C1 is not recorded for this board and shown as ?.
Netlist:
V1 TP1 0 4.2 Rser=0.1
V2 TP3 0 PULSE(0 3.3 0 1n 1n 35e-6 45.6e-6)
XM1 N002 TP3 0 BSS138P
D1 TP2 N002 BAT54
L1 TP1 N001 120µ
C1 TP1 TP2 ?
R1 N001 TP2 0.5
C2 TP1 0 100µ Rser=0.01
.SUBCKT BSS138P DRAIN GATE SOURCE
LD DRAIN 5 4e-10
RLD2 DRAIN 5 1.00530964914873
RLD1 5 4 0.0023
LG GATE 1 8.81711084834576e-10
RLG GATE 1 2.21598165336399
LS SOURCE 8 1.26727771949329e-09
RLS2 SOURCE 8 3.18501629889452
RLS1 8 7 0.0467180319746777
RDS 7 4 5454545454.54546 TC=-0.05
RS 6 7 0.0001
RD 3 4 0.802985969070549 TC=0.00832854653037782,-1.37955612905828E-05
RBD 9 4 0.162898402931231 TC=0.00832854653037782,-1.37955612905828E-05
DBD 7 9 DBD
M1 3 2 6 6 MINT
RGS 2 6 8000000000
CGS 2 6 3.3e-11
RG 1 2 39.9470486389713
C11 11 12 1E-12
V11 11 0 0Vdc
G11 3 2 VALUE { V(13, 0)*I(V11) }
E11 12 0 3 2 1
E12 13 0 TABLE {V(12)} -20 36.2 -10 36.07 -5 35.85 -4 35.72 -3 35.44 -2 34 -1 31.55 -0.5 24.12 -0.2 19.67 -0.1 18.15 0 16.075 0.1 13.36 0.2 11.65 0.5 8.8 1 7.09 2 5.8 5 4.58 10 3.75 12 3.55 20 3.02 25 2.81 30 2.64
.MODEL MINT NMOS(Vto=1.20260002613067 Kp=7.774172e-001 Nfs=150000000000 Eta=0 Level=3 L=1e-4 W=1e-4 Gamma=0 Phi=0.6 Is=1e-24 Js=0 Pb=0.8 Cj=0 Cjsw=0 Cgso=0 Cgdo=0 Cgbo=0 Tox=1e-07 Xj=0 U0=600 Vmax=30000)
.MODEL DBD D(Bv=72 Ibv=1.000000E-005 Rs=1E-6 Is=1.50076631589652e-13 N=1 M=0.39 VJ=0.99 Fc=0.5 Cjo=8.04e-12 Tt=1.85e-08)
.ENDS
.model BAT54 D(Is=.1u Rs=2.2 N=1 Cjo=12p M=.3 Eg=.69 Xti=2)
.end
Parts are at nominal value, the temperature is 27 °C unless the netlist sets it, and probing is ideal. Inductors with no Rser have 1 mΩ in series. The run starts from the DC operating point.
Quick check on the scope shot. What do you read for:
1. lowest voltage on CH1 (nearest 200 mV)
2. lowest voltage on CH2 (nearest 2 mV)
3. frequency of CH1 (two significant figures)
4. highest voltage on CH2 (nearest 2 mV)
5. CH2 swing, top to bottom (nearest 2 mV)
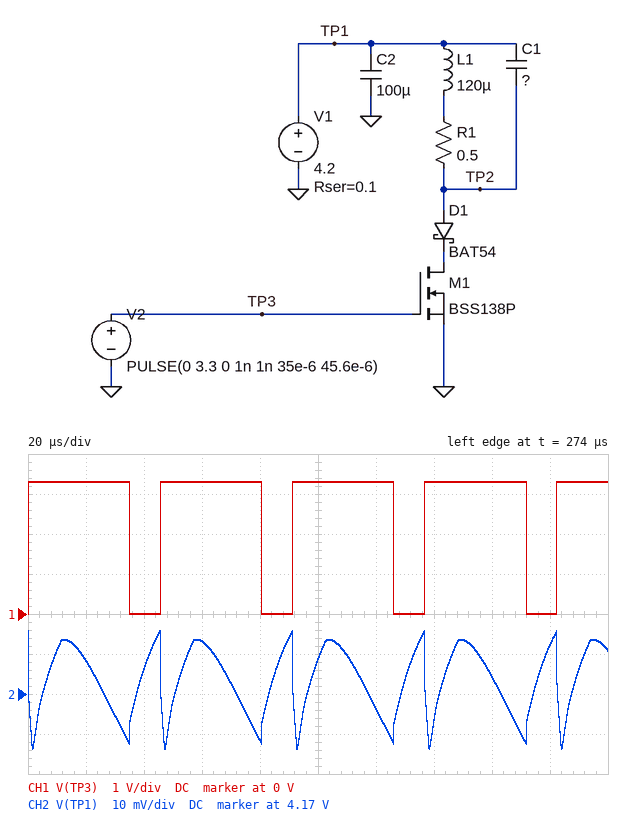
0 V
4.156 V
22 kHz
4.186 V
30 mV
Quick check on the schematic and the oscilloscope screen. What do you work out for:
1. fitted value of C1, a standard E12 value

270 nF
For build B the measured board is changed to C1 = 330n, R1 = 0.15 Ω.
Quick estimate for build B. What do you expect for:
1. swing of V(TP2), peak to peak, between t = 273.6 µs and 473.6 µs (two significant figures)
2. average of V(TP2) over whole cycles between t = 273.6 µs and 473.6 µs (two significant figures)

15 V
4.1 V
